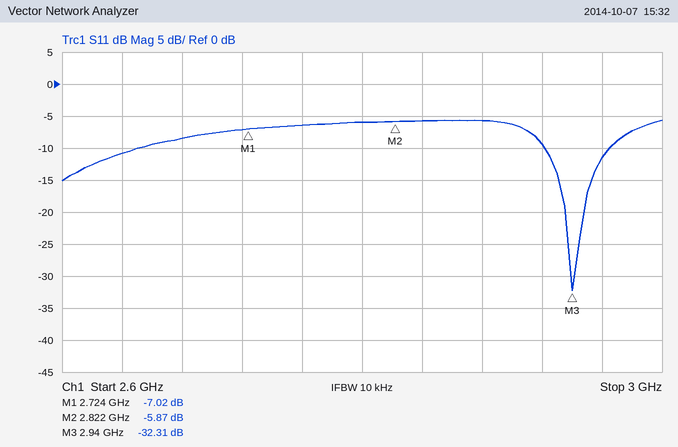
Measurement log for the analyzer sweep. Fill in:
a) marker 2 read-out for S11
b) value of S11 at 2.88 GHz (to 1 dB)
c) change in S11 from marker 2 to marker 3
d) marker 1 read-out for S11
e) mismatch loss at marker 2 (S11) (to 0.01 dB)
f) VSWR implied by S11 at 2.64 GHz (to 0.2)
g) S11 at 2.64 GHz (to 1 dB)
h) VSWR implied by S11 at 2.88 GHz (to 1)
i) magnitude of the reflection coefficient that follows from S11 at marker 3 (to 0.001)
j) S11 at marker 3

-5.87 dB
-6 dB
-26.44 dB
-7.02 dB
1.30 dB
1.8
-11 dB
3
0.024
-32.31 dB
